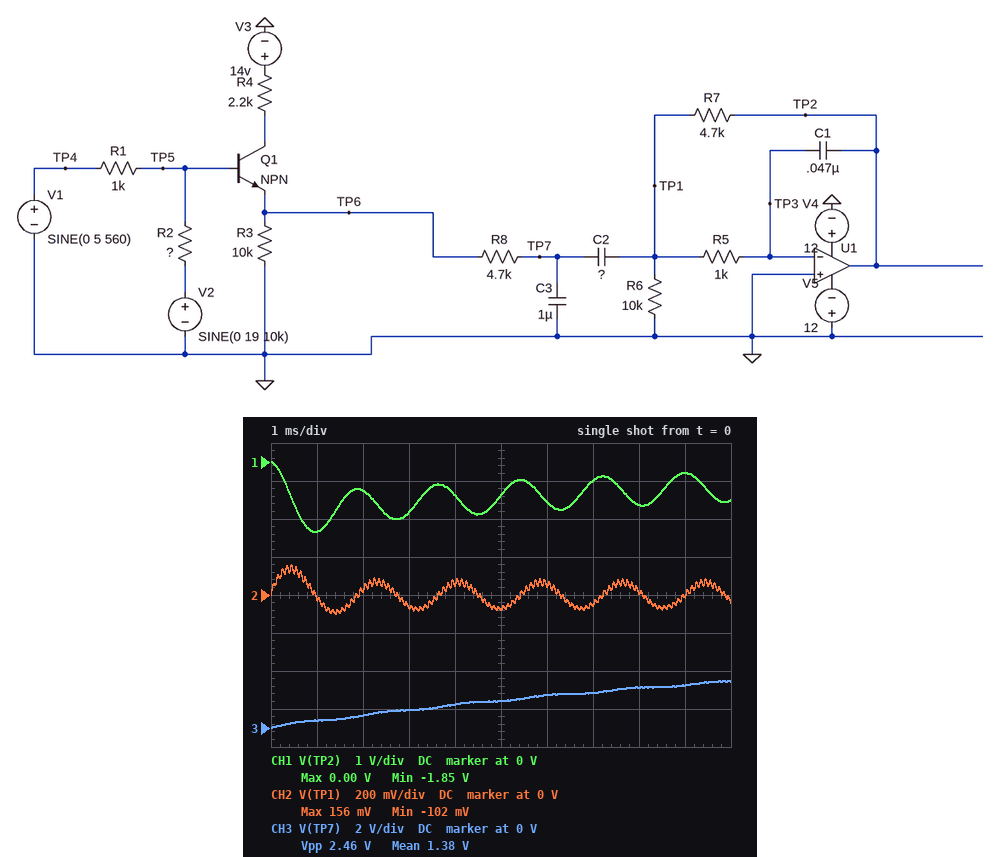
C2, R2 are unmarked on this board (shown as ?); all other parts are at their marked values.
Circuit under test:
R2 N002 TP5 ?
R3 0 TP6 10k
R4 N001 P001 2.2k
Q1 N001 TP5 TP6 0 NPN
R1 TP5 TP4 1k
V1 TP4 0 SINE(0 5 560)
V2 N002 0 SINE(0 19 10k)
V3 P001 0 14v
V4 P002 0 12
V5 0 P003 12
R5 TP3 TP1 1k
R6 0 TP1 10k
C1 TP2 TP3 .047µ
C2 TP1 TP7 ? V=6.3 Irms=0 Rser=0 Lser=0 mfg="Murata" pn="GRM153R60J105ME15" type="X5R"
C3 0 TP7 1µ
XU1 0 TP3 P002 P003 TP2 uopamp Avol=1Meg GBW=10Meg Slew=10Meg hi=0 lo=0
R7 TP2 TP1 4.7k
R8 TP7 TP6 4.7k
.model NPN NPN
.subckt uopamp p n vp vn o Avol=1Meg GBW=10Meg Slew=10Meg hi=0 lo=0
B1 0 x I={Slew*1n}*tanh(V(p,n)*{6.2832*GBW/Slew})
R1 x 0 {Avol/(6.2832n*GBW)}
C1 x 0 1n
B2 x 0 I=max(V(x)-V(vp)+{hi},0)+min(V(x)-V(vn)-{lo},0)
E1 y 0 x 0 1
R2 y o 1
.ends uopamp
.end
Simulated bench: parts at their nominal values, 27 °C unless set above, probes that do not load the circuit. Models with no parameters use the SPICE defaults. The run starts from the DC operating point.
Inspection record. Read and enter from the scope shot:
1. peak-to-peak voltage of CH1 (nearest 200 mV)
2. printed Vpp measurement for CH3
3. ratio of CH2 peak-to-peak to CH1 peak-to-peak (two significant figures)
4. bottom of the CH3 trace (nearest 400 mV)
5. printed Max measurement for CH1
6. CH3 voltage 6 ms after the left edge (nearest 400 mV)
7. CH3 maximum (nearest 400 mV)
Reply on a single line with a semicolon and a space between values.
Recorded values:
1.8 V; 2.46 V; 0.14; 0 V; 0.00 V; 1.6 V; 2.4 V
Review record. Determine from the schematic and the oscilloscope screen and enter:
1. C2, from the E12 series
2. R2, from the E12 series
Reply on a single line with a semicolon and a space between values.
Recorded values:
820 nF; 820 Ω
